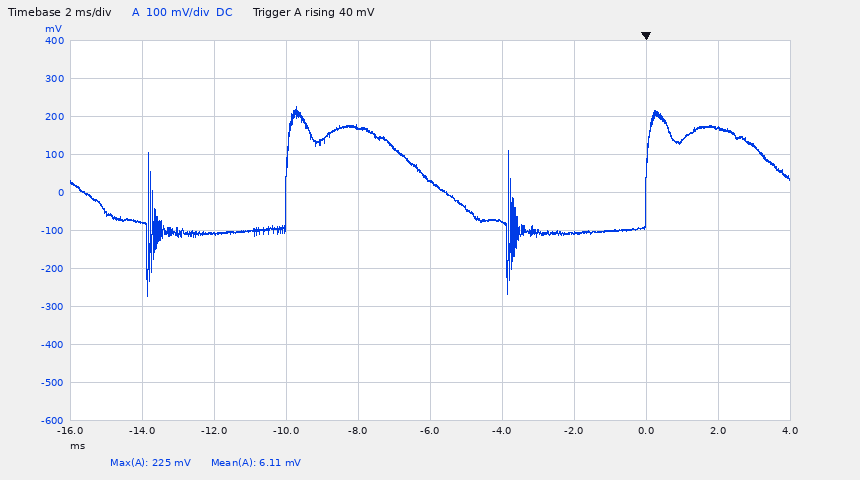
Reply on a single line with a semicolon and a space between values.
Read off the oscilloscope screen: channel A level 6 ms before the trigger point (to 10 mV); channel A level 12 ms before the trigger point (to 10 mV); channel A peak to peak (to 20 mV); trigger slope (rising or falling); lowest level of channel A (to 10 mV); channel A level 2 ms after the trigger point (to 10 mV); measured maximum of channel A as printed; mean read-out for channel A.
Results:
30 mV; -110 mV; 500 mV; rising; -270 mV; 170 mV; 225 mV; 6.11 mV
